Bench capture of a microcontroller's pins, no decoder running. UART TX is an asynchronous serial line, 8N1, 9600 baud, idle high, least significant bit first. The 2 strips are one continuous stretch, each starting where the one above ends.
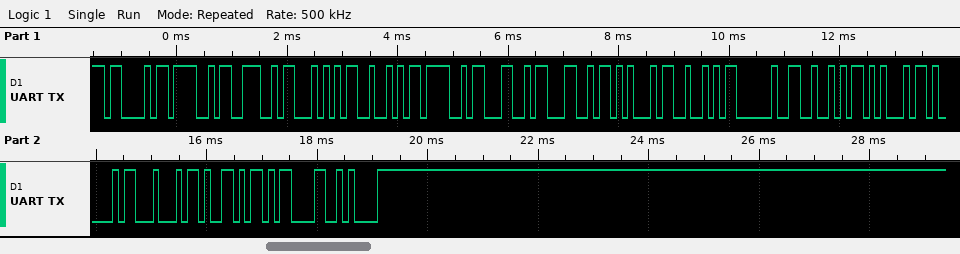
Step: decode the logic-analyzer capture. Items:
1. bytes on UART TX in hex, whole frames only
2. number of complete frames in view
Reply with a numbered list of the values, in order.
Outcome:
1. 0x43 0x4F 0x4E 0x54 0x52 0x4F 0x4C 0x4C 0x45 0x52 0x20 0x52 0x45 0x41 0x44 0x59 0x0D 0x0A
2. 18
